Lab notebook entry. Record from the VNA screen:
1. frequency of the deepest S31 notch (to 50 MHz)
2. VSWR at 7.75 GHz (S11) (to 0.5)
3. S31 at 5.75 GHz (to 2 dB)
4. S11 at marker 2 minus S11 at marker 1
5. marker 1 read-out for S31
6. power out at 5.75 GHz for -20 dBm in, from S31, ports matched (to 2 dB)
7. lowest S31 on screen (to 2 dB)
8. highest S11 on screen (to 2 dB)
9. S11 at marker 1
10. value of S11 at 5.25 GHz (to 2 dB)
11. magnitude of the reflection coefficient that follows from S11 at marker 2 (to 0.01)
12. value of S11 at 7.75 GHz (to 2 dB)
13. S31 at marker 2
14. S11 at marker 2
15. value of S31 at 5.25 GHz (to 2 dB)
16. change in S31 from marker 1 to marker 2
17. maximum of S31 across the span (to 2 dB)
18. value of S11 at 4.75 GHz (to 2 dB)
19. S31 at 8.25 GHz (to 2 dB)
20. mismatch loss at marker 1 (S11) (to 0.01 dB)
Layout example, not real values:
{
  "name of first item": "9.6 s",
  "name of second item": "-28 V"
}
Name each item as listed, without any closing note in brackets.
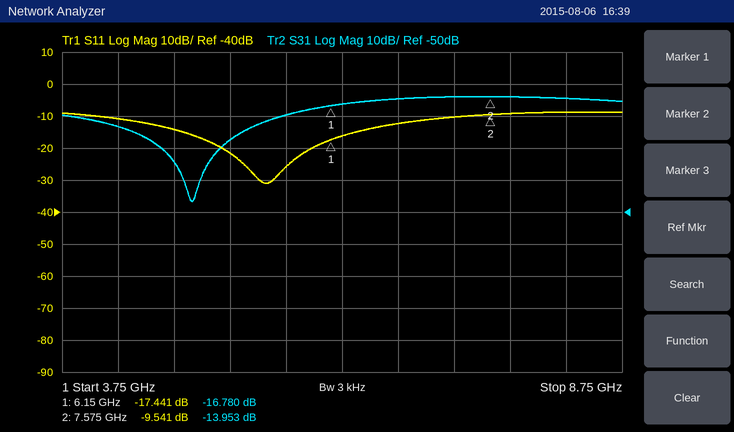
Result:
{
  "frequency of the deepest S31 notch": "4.90 GHz",
  "VSWR at 7.75 GHz (S11)": "2.0",
  "S31 at 5.75 GHz": "-20 dB",
  "S11 at marker 2 minus S11 at marker 1": "7.900 dB",
  "marker 1 read-out for S31": "-16.780 dB",
  "power out at 5.75 GHz for -20 dBm in, from S31, ports matched": "-40 dBm",
  "lowest S31 on screen": "-46 dB",
  "highest S11 on screen": "-8 dB",
  "S11 at marker 1": "-17.441 dB",
  "value of S11 at 5.25 GHz": "-22 dB",
  "magnitude of the reflection coefficient that follows from S11 at marker 2": "0.33",
  "value of S11 at 7.75 GHz": "-10 dB",
  "S31 at marker 2": "-13.953 dB",
  "S11 at marker 2": "-9.541 dB",
  "value of S31 at 5.25 GHz": "-28 dB",
  "change in S31 from marker 1 to marker 2": "2.827 dB",
  "maximum of S31 across the span": "-14 dB",
  "value of S11 at 4.75 GHz": "-14 dB",
  "S31 at 8.25 GHz": "-14 dB",
  "mismatch loss at marker 1 (S11)": "0.08 dB"
}
